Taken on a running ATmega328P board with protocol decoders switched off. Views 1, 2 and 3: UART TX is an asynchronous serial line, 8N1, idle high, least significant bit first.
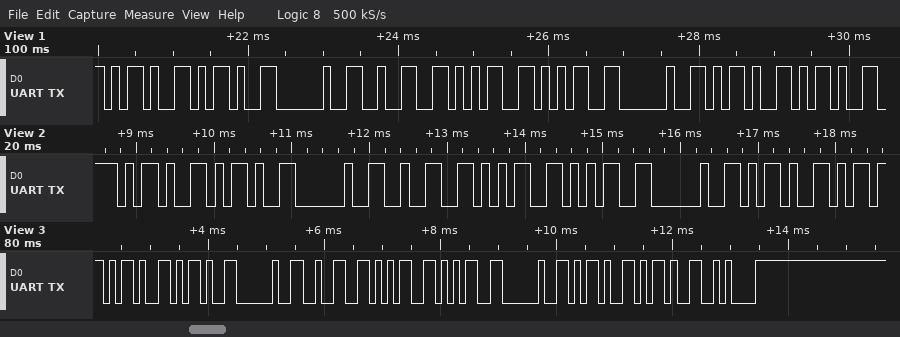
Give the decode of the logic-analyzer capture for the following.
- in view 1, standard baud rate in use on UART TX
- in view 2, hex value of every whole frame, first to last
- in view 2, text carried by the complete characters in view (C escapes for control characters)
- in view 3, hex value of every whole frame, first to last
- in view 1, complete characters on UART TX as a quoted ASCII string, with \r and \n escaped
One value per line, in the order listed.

9600 baud
2D 2D 20 32 35 35 20 2D
"-- 255 -"
2D 2D 20 32 35 35 20 2D 2D 0A
"-- 255 --"
